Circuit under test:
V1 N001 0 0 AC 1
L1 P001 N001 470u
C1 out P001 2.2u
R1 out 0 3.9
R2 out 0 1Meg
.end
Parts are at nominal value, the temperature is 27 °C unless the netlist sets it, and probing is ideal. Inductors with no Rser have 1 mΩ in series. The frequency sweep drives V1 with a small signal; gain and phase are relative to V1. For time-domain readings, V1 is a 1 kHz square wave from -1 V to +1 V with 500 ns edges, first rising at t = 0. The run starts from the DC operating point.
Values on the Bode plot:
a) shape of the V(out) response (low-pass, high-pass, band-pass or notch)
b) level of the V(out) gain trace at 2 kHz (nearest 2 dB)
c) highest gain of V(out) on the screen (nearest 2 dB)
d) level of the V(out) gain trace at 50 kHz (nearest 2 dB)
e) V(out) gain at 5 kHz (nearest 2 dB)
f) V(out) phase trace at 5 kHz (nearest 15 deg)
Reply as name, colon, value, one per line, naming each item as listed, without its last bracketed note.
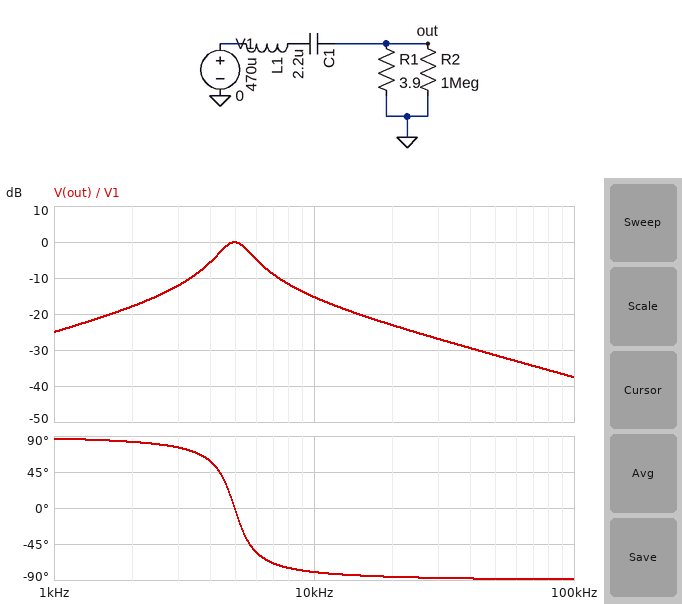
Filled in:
shape of the V(out) response: band-pass
level of the V(out) gain trace at 2 kHz: -18 dB
highest gain of V(out) on the screen: 0 dB
level of the V(out) gain trace at 50 kHz: -32 dB
V(out) gain at 5 kHz: 0 dB
V(out) phase trace at 5 kHz: 0 deg
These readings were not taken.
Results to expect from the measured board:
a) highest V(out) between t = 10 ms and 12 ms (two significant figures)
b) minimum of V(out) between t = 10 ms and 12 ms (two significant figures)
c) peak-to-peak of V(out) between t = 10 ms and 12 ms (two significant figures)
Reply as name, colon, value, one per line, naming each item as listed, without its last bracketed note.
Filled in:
highest V(out) between t = 10 ms and 12 ms: 500 mV
minimum of V(out) between t = 10 ms and 12 ms: -500 mV
peak-to-peak of V(out) between t = 10 ms and 12 ms: 990 mV
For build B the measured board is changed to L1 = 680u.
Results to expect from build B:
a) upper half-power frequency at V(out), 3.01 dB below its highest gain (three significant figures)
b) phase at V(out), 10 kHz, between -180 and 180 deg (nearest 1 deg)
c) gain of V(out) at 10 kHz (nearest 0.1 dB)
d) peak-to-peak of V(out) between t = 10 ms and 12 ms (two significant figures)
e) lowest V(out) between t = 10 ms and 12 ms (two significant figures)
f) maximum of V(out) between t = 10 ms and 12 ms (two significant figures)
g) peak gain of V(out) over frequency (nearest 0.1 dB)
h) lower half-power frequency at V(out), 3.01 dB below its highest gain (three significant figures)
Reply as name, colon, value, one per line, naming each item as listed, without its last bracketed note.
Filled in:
upper half-power frequency at V(out), 3.01 dB below its highest gain: 4.60 kHz
phase at V(out), 10 kHz, between -180 and 180 deg: -84 deg
gain of V(out) at 10 kHz: -19.2 dB
peak-to-peak of V(out) between t = 10 ms and 12 ms: 610 mV
lowest V(out) between t = 10 ms and 12 ms: -300 mV
maximum of V(out) between t = 10 ms and 12 ms: 300 mV
peak gain of V(out) over frequency: 0 dB
lower half-power frequency at V(out), 3.01 dB below its highest gain: 3.68 kHz
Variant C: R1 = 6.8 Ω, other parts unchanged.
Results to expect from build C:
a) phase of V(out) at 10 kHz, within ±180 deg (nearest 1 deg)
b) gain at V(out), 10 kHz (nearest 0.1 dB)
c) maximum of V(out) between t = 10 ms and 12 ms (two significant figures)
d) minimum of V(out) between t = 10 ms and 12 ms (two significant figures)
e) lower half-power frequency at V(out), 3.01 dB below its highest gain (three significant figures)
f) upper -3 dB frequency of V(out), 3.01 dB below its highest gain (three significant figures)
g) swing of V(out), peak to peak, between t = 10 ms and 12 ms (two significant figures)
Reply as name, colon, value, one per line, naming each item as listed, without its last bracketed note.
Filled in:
phase of V(out) at 10 kHz, within ±180 deg: -73 deg
gain at V(out), 10 kHz: -10.7 dB
maximum of V(out) between t = 10 ms and 12 ms: 690 mV
minimum of V(out) between t = 10 ms and 12 ms: -690 mV
lower half-power frequency at V(out), 3.01 dB below its highest gain: 3.93 kHz
upper -3 dB frequency of V(out), 3.01 dB below its highest gain: 6.23 kHz
swing of V(out), peak to peak, between t = 10 ms and 12 ms: 1.4 V
